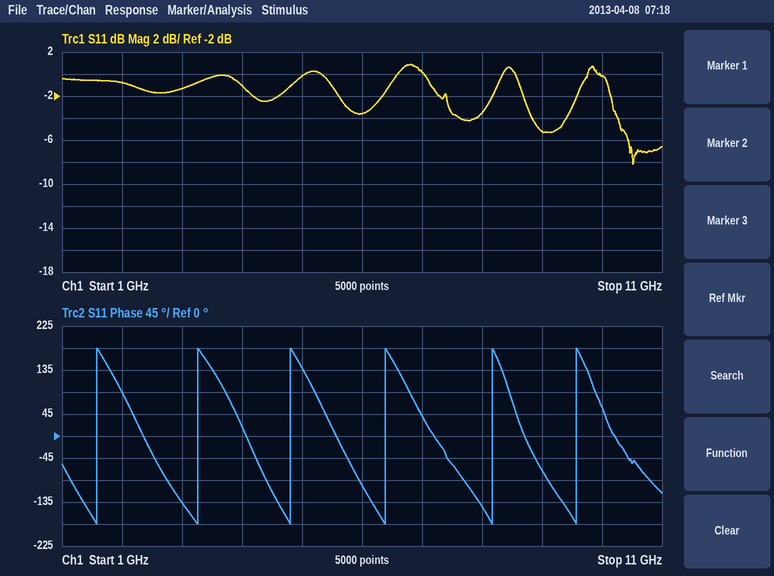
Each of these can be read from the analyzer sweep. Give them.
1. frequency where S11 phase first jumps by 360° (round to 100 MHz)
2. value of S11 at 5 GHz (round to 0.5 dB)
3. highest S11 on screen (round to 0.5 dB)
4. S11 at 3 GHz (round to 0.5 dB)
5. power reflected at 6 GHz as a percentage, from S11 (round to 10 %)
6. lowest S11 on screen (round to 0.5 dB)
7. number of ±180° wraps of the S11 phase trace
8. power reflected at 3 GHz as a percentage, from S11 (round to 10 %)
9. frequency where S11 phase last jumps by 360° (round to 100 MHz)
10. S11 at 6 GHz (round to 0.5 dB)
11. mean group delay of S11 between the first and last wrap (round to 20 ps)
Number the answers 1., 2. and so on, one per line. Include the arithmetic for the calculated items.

1. 1.6 GHz
2. 0.0 dB
3. 1.0 dB
4. -1.5 dB
5. 10^(-3.5/10) ≈ 44.7 %, so 40 % to the nearest 10 %
6. -8.0 dB
7. 6
8. 10^(-1.5/10) ≈ 70.8 %, so 70 % to the nearest 10 %
9. 9.6 GHz
10. -3.5 dB
11. 5 cycles / (9.6 GHz − 1.6 GHz) ≈ 625 ps, so 620 ps to the nearest 20 ps
